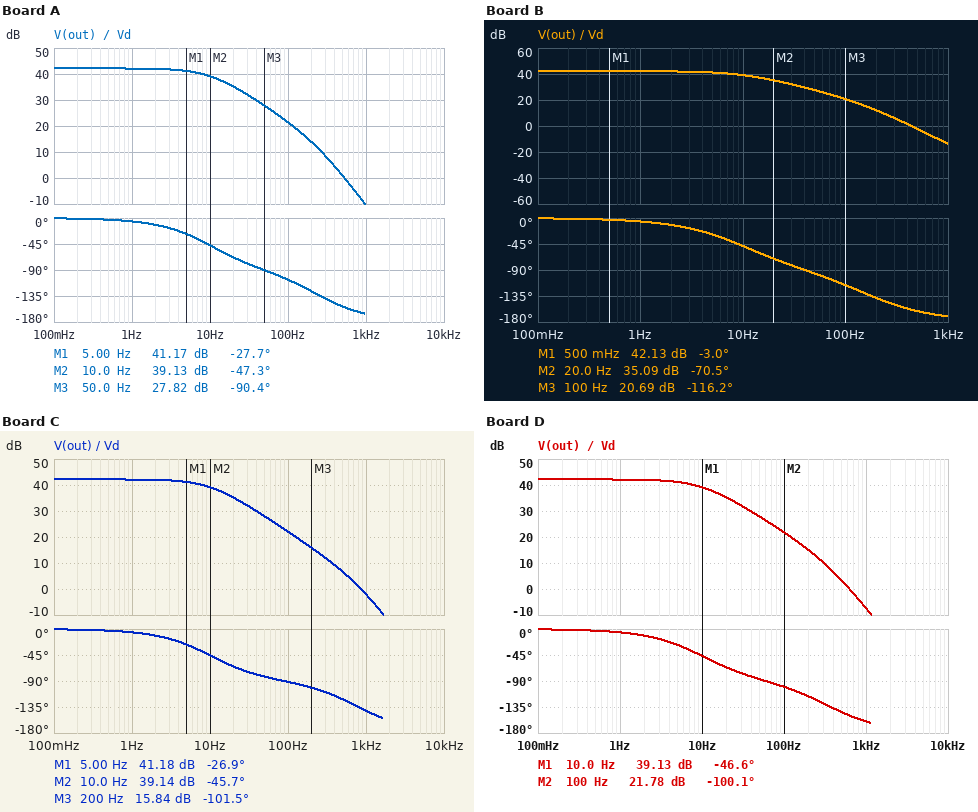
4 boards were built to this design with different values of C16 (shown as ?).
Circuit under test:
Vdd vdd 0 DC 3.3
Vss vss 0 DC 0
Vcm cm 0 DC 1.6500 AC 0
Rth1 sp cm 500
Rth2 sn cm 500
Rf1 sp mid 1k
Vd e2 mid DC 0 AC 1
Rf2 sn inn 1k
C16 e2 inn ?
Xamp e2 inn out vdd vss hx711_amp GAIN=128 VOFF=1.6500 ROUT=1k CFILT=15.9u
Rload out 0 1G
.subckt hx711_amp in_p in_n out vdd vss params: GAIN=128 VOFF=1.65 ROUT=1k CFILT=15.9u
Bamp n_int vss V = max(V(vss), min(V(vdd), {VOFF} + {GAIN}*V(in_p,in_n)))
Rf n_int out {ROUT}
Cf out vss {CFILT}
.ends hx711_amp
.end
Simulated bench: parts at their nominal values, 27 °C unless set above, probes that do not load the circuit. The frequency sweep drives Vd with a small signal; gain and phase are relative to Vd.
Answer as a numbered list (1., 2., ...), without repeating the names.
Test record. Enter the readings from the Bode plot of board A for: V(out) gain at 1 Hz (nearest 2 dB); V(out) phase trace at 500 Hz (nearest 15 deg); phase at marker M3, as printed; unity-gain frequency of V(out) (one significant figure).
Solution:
1. 42 dB
2. -150 deg
3. -90.4 deg
4. 500 Hz
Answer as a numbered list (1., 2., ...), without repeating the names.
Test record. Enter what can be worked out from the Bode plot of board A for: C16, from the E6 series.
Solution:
1. 220 nF
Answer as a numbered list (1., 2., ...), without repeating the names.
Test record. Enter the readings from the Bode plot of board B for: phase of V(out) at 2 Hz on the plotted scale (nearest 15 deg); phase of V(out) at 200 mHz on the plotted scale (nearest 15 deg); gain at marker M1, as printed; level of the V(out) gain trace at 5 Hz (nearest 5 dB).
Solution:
1. -15 deg
2. 0 deg
3. 42.13 dB
4. 40 dB
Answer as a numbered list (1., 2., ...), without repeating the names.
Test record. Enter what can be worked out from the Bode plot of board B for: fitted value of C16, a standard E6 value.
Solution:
1. 330 nF
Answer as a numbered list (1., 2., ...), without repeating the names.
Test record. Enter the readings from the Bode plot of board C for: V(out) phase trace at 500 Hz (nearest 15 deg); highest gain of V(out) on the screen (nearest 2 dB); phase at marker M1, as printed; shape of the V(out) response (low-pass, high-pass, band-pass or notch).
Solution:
1. -120 deg
2. 42 dB
3. -26.9 deg
4. low-pass
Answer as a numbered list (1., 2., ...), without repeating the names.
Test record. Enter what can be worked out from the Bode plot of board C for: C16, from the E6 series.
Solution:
1. 68 nF
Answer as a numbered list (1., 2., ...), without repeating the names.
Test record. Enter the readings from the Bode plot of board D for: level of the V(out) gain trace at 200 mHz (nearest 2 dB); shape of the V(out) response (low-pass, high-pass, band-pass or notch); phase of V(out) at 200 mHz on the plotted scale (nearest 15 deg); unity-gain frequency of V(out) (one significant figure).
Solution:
1. 42 dB
2. low-pass
3. 0 deg
4. 600 Hz
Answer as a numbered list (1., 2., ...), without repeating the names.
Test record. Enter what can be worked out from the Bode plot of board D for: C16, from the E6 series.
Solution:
1. 150 nF
